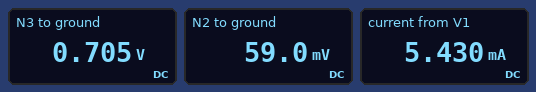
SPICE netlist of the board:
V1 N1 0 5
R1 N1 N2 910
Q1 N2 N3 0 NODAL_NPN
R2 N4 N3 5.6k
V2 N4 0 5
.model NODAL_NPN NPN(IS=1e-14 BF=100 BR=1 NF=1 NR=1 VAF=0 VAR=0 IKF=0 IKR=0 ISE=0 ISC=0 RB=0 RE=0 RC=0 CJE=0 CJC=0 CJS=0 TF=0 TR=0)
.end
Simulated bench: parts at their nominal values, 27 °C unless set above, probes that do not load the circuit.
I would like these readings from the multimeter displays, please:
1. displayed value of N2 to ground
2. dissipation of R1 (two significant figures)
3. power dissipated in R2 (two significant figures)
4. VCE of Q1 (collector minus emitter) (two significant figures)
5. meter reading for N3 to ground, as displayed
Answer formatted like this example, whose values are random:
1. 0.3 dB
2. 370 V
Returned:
1. 59.0 mV
2. 27 mW
3. 3.3 mW
4. 59 mV
5. 0.705 V
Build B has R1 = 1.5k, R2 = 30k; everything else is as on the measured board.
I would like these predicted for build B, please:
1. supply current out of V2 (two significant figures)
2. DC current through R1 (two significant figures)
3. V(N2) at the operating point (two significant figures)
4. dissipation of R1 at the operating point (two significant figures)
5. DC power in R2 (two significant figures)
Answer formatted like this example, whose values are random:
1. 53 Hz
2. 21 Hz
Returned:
1. 140 µA
2. 3.3 mA
3. 90 mV
4. 16 mW
5. 620 µW
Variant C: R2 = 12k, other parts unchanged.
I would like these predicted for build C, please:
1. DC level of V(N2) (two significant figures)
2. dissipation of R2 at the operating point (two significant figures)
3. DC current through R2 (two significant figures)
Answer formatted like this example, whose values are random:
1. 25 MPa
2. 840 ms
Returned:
1. 78 mV
2. 1.5 mW
3. 360 µA
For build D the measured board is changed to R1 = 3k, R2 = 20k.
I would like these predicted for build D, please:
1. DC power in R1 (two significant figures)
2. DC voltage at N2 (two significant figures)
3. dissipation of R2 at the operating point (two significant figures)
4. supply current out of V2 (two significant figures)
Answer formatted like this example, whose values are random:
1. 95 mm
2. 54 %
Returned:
1. 8.1 mW
2. 61 mV
3. 940 µW
4. 220 µA
